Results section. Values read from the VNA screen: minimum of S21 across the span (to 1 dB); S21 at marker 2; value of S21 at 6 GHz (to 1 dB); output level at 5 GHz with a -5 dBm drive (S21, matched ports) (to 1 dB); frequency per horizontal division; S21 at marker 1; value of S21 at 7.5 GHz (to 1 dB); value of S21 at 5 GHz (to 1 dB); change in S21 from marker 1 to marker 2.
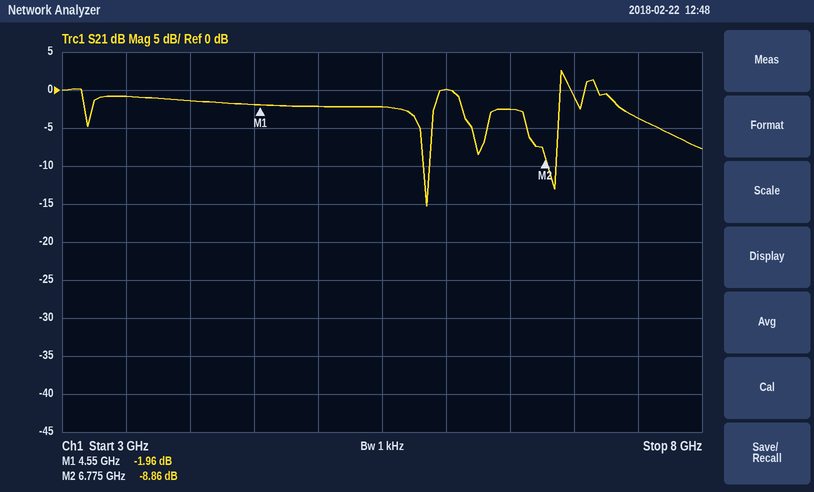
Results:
-15 dB
-8.86 dB
0 dB
-7 dBm
500 MHz
-1.96 dB
-4 dB
-2 dB
-6.90 dB
